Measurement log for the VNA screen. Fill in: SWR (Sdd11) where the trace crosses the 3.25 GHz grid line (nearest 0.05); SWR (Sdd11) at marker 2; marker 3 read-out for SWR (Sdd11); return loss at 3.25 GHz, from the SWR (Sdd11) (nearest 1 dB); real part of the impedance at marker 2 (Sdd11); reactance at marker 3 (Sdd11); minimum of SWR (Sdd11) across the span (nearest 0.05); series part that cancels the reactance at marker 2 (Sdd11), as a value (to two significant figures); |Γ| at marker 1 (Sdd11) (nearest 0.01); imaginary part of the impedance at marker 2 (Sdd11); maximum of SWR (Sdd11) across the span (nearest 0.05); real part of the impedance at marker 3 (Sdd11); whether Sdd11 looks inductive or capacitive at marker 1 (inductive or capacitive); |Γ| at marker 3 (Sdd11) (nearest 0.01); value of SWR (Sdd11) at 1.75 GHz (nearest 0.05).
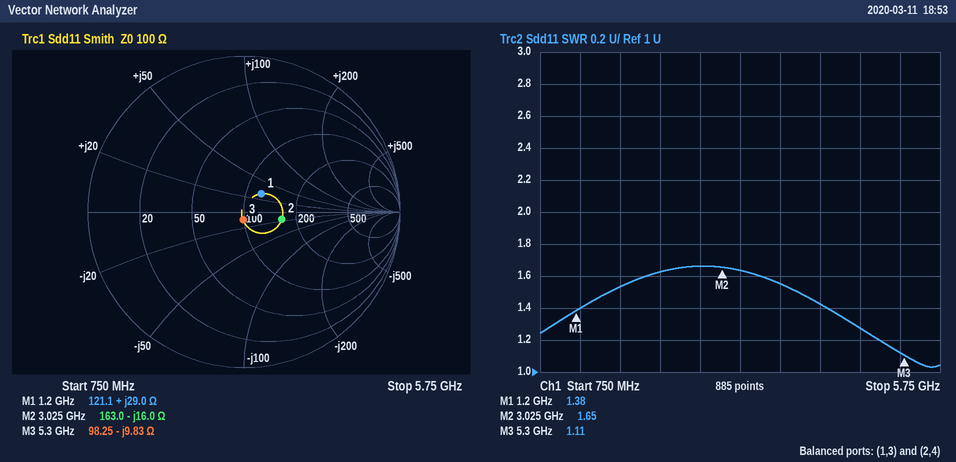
1.65
1.65
1.11
12 dB
163.0 Ω
-9.83 Ω
1.05
840 pH
0.16
-16.0 Ω
1.65
98.25 Ω
inductive
0.05
1.55
